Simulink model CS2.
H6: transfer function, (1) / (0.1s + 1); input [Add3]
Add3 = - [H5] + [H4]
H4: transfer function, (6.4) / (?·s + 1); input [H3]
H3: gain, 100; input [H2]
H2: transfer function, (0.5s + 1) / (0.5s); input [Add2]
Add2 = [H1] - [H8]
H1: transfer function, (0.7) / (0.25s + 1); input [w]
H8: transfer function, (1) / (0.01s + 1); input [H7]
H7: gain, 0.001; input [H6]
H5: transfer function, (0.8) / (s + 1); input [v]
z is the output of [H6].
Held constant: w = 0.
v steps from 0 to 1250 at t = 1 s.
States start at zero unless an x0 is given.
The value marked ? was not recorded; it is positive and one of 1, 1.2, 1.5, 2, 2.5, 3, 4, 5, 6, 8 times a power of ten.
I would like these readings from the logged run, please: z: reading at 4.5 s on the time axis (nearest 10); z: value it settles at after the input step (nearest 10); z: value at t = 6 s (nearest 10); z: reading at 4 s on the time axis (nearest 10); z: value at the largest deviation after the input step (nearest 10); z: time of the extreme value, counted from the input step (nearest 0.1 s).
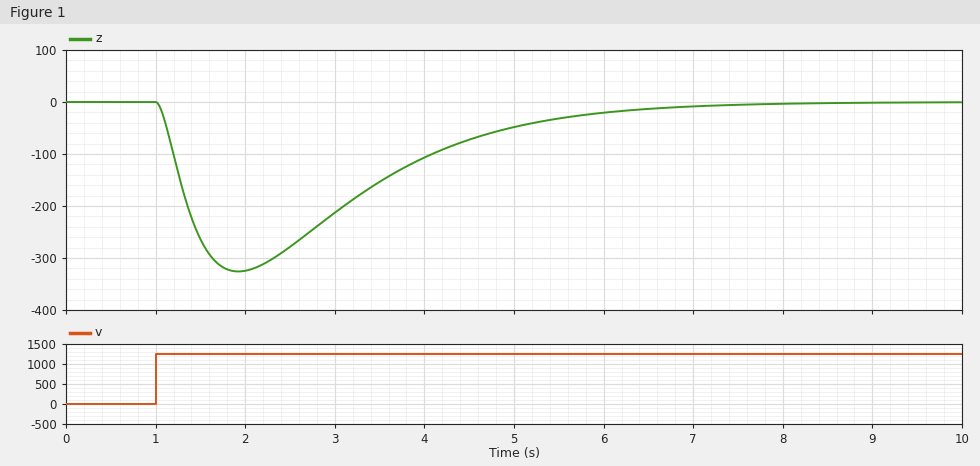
-70
0
-20
-110
-330
0.9 s
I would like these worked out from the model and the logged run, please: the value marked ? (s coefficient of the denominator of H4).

0.4
